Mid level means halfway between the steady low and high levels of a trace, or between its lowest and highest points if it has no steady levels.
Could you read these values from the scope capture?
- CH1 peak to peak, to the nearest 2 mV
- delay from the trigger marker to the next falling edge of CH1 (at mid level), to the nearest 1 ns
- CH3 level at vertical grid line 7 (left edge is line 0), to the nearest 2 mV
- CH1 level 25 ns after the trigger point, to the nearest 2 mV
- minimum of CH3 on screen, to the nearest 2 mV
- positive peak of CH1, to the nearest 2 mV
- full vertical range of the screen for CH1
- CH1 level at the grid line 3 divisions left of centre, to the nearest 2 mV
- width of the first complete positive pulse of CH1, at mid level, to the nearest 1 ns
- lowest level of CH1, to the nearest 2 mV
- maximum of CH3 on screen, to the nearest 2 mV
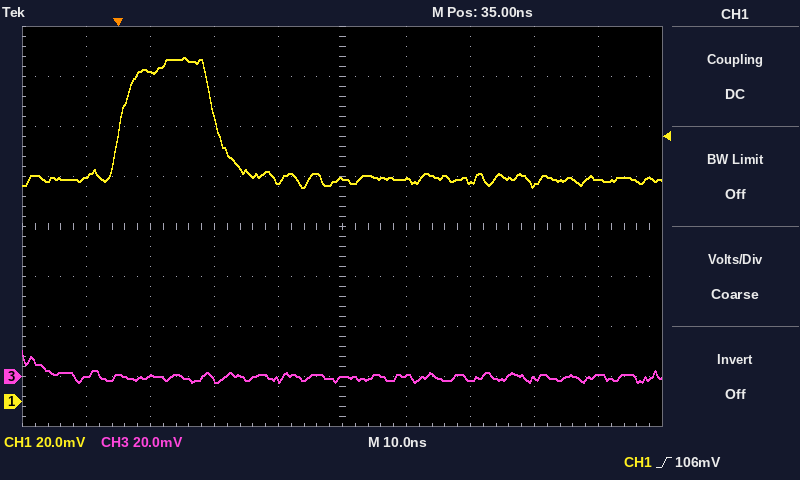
52 mV
15 ns
-2 mV
88 mV
-2 mV
138 mV
160 mV
132 mV
15 ns
86 mV
10 mV
